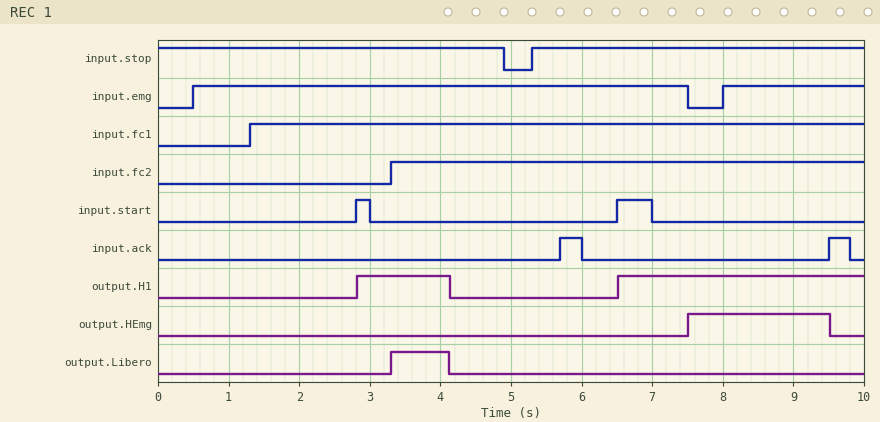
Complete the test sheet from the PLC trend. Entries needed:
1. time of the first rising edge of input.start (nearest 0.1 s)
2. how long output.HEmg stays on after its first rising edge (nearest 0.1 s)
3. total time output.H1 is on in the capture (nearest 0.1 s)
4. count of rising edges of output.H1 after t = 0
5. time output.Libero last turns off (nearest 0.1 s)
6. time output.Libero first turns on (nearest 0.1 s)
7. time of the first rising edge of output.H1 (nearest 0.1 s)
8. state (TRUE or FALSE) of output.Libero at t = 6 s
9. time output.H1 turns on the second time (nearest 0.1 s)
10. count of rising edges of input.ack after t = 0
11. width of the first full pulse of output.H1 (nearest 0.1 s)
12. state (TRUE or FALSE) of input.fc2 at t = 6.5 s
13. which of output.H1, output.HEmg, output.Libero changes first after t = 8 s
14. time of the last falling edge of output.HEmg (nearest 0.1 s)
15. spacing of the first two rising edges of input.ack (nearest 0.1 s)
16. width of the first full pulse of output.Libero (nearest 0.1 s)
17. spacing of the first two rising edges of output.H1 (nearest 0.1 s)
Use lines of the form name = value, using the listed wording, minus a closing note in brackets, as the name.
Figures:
time of the first rising edge of input.start = 2.8 s
how long output.HEmg stays on after its first rising edge = 2.0 s
total time output.H1 is on in the capture = 4.8 s
count of rising edges of output.H1 after t = 0 = 2
time output.Libero last turns off = 4.1 s
time output.Libero first turns on = 3.3 s
time of the first rising edge of output.H1 = 2.8 s
state (TRUE or FALSE) of output.Libero at t = 6 s = FALSE
time output.H1 turns on the second time = 6.5 s
count of rising edges of input.ack after t = 0 = 2
width of the first full pulse of output.H1 = 1.3 s
state (TRUE or FALSE) of input.fc2 at t = 6.5 s = TRUE
which of output.H1, output.HEmg, output.Libero changes first after t = 8 s = output.HEmg
time of the last falling edge of output.HEmg = 9.5 s
spacing of the first two rising edges of input.ack = 3.8 s
width of the first full pulse of output.Libero = 0.8 s
spacing of the first two rising edges of output.H1 = 3.7 s
